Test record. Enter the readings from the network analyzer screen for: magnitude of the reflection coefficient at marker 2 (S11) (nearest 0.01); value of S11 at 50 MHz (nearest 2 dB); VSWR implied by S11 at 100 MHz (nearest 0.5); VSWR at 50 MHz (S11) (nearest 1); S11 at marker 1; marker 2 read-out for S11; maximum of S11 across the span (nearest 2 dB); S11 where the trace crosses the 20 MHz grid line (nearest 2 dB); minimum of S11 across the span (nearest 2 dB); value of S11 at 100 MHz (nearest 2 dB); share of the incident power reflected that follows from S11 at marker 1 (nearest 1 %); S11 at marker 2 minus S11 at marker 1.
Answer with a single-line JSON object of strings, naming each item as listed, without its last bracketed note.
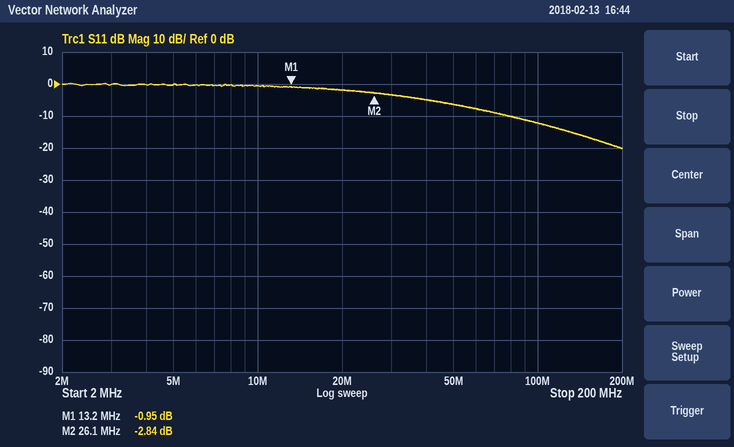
{"magnitude of the reflection coefficient at marker 2 (S11)": "0.72", "value of S11 at 50 MHz": "-6 dB", "VSWR implied by S11 at 100 MHz": "1.5", "VSWR at 50 MHz (S11)": "3", "S11 at marker 1": "-0.95 dB", "marker 2 read-out for S11": "-2.84 dB", "maximum of S11 across the span": "0 dB", "S11 where the trace crosses the 20 MHz grid line": "-2 dB", "minimum of S11 across the span": "-20 dB", "value of S11 at 100 MHz": "-12 dB", "share of the incident power reflected that follows from S11 at marker 1": "80 %", "S11 at marker 2 minus S11 at marker 1": "-1.89 dB"}
